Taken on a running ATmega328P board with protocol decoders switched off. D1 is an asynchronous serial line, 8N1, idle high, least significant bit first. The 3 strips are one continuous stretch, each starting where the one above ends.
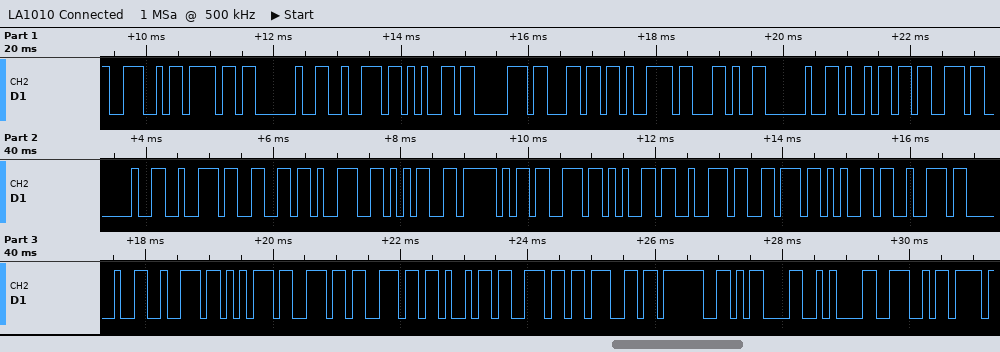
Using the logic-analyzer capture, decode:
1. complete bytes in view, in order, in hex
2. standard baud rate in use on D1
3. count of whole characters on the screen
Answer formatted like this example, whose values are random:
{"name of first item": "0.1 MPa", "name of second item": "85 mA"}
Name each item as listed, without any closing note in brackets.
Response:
{"complete bytes in view, in order, in hex": "4E 6F 20 72 65 70 6C 79 2C 20 69 73 20 72 66 39 35 5F 73 65 72 76 65 72 20 72 75 6E 6E 69 6E 67 3F 0D 0A 4E", "standard baud rate in use on D1": "9600 baud", "count of whole characters on the screen": "36"}
